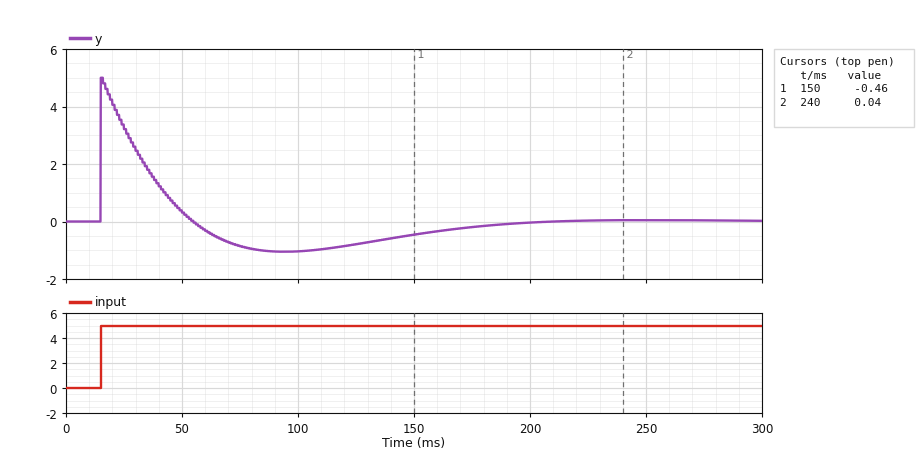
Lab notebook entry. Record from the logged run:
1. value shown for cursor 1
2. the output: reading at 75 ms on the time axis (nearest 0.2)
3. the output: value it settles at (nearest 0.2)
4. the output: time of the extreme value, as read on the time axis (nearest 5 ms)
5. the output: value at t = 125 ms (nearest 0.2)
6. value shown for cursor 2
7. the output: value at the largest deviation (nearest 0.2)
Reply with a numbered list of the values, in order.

1. -0.46
2. -0.8
3. 0.0
4. 15 ms
5. -0.8
6. 0.04
7. 5.0
